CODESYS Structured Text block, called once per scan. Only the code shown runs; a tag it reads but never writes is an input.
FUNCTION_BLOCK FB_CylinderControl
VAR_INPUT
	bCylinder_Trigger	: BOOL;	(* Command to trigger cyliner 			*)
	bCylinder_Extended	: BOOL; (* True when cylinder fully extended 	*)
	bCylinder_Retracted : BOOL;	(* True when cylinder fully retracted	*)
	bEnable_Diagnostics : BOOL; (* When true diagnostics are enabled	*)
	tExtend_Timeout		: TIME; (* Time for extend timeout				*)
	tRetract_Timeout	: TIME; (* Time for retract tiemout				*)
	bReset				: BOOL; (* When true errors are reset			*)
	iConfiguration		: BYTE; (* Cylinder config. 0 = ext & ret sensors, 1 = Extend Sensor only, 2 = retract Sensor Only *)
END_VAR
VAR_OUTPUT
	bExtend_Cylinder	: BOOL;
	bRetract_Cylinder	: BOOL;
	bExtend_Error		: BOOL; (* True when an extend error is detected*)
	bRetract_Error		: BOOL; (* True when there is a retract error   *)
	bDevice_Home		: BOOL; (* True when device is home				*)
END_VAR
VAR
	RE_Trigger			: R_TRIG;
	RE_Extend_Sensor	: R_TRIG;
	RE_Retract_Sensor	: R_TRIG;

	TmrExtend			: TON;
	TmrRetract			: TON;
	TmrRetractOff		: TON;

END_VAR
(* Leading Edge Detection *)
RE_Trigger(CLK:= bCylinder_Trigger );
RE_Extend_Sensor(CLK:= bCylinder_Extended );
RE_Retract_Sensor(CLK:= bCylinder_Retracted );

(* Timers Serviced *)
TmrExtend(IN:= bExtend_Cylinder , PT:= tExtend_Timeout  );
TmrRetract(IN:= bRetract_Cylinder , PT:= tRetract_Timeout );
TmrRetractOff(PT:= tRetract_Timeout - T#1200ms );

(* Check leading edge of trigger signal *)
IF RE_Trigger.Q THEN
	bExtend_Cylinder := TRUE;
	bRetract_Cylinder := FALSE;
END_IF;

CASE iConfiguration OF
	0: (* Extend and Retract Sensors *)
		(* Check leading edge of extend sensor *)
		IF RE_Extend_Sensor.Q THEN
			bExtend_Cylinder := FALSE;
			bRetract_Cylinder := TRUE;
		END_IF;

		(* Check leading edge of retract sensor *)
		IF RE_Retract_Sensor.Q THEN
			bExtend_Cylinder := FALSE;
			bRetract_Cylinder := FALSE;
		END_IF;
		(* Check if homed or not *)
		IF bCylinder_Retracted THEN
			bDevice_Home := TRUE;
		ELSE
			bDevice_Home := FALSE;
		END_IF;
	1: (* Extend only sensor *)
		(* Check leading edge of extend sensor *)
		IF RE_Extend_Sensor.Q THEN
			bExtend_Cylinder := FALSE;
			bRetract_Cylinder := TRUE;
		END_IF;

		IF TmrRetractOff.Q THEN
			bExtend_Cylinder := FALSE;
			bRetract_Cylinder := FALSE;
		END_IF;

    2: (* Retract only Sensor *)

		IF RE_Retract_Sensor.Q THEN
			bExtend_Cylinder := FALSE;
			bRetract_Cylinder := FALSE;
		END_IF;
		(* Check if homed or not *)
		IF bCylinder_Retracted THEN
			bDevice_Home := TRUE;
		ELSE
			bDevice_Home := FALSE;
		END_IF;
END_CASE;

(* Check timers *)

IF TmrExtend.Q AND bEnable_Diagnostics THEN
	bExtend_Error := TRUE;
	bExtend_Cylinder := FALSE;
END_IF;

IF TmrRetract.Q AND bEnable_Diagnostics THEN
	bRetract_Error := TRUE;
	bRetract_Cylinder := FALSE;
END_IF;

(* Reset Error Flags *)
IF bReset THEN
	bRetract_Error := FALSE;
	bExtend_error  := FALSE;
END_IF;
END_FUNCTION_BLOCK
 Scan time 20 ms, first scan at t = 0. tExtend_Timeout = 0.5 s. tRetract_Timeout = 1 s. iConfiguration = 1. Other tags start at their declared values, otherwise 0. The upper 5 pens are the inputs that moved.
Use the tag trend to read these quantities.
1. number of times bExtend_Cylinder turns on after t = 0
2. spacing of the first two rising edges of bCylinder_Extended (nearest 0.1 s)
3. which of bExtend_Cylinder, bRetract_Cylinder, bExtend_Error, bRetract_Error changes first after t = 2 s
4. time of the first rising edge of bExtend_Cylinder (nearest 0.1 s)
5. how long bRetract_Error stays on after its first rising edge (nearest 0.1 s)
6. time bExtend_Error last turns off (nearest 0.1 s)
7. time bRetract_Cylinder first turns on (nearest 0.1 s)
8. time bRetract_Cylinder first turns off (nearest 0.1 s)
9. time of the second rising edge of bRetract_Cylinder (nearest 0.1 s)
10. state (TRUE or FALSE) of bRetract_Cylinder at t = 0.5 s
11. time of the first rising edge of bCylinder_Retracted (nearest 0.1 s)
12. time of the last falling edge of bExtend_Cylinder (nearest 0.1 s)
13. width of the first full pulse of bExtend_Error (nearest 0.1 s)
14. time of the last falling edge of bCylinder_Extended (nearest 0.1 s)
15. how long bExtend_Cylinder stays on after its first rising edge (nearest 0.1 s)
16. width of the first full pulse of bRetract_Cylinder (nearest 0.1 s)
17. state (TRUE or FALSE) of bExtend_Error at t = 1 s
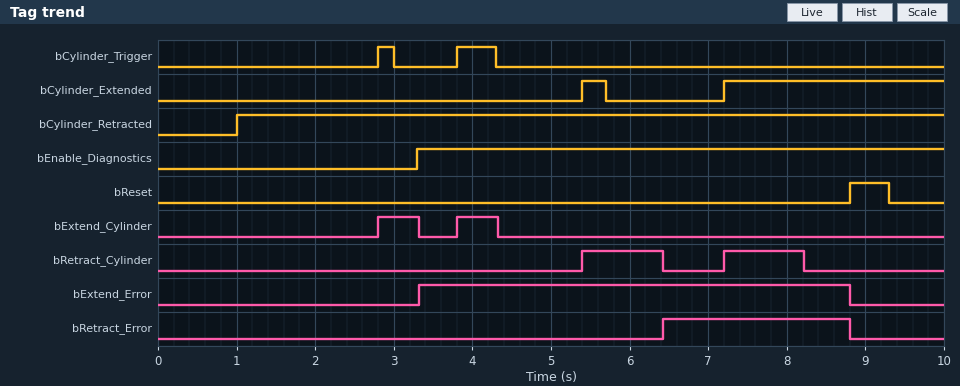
2
1.8 s
bExtend_Cylinder
2.8 s
2.4 s
8.8 s
5.4 s
6.4 s
7.2 s
FALSE
1.0 s
4.3 s
5.5 s
5.7 s
0.5 s
1.0 s
FALSE
